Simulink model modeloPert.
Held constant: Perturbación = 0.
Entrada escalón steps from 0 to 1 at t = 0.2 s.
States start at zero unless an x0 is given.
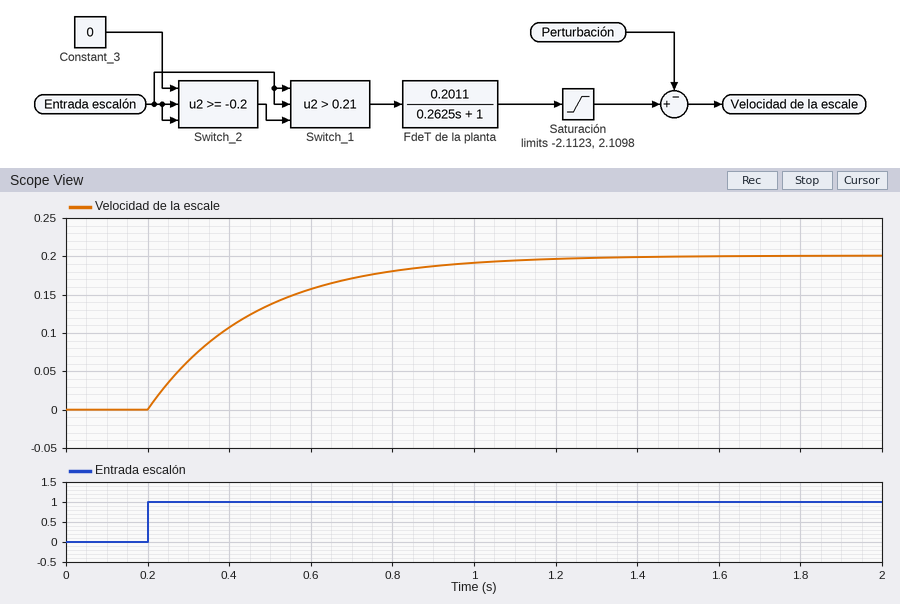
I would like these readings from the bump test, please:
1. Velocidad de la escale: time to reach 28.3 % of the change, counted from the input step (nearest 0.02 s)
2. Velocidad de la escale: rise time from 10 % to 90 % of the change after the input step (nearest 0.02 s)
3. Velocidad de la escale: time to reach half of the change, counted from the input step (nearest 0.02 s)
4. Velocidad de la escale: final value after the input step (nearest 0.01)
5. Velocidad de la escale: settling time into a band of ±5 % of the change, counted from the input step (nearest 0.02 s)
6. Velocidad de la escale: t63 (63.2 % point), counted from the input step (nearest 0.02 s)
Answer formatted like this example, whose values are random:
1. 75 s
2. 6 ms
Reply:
1. 0.08 s
2. 0.58 s
3. 0.18 s
4. 0.20
5. 0.78 s
6. 0.26 s
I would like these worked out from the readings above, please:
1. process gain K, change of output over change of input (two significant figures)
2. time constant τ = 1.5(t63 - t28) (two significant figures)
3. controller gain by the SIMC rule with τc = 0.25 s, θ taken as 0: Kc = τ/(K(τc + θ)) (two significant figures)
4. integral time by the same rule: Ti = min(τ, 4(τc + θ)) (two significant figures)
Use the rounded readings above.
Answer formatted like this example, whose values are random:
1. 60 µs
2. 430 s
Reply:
1. 0.20
2. 0.27 s
3. 5.4
4. 0.27 s
